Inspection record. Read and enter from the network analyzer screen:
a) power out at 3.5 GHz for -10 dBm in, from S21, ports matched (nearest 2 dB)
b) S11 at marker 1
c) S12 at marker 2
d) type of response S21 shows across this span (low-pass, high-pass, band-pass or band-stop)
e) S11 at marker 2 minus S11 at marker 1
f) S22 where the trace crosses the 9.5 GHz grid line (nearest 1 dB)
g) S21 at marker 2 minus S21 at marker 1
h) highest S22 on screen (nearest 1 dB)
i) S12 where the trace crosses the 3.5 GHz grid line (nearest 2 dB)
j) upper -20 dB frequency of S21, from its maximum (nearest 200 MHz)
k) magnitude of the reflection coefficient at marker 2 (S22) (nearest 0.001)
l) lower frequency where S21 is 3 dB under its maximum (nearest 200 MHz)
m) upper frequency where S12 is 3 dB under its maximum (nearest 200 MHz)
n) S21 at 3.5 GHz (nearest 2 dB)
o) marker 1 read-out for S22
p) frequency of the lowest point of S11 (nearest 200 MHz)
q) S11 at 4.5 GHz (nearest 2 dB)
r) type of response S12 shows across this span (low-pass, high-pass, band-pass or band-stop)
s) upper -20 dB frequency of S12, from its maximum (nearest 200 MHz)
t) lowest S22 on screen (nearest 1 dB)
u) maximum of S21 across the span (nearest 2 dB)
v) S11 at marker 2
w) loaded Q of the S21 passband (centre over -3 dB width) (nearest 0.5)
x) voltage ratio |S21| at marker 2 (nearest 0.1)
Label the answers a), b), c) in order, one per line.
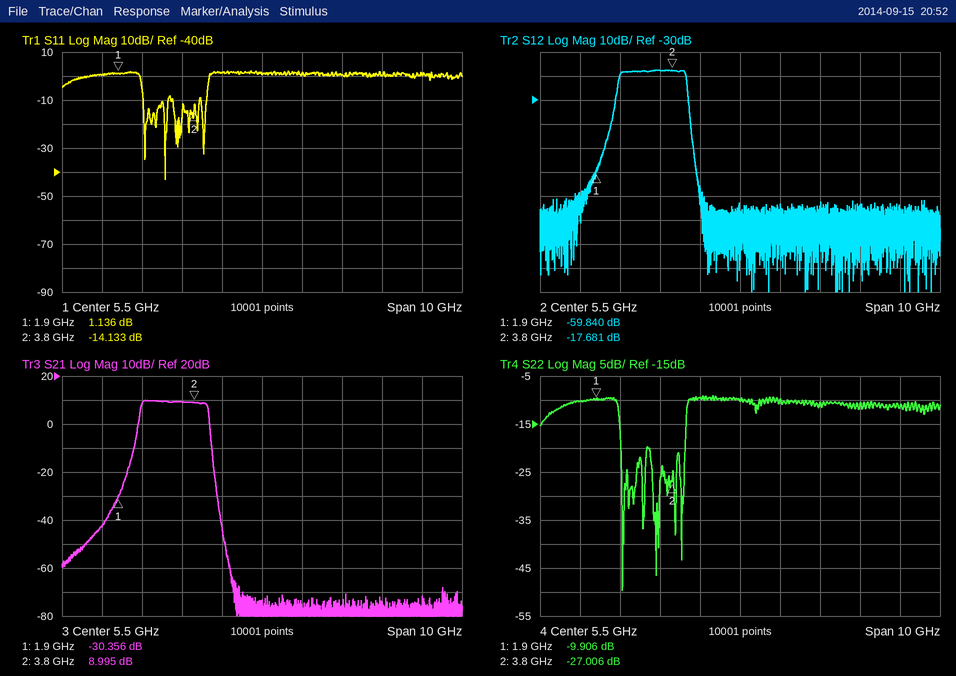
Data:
a) 0 dBm
b) 1.136 dB
c) -17.681 dB
d) band-pass
e) -15.269 dB
f) -11 dB
g) 39.351 dB
h) -9 dB
i) -18 dB
j) 4.2 GHz
k) 0.045
l) 2.4 GHz
m) 4.2 GHz
n) 10 dB
o) -9.906 dB
p) 3.0 GHz
q) 2 dB
r) band-pass
s) 4.2 GHz
t) -50 dB
u) 10 dB
v) -14.133 dB
w) 2.0
x) 2.8
